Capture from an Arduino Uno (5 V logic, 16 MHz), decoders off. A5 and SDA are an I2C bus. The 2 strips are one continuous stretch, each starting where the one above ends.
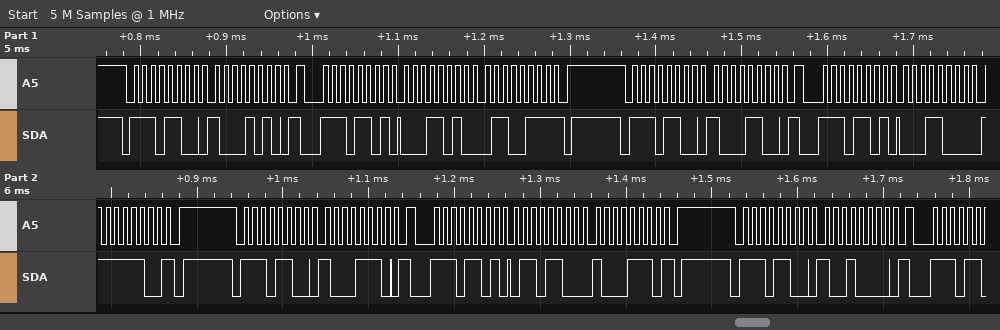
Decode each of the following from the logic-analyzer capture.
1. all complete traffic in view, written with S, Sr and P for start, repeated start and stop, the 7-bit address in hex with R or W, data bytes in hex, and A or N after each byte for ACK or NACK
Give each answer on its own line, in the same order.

S 76W A 8A A Sr 76R A 1A A 67 N P S 76W A 8C A Sr 76R A 18 A FC N P S 76W A 8E A Sr 76R A 6C A 8E N P S 76W A 90 A
